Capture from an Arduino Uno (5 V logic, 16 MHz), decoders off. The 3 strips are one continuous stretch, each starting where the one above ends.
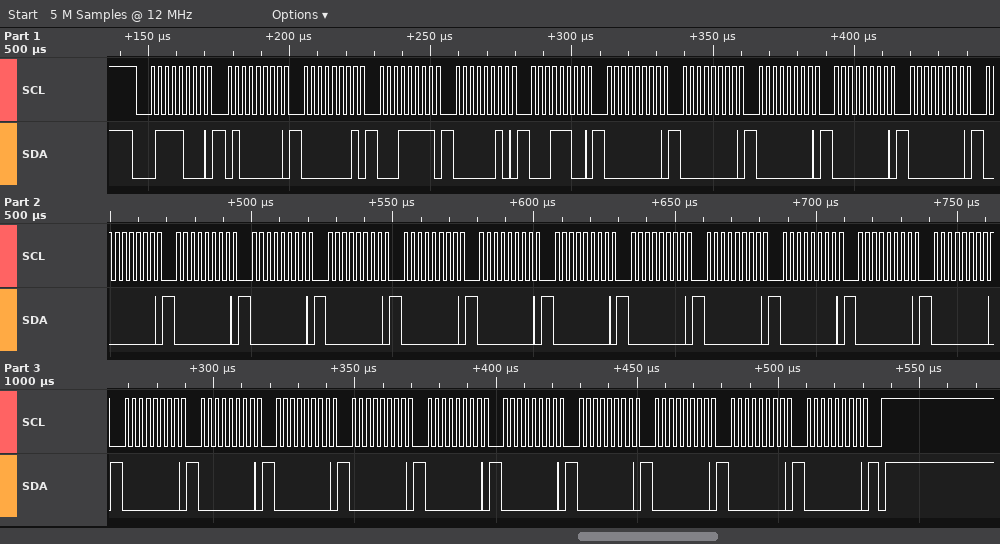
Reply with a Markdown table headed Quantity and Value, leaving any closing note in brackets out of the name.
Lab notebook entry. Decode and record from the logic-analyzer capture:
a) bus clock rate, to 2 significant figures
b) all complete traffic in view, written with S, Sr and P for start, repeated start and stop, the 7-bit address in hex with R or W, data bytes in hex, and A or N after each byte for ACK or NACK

| Quantity | Value |
|---|---|
| bus clock rate, to 2 significant figures | 400 kHz |
| all complete traffic in view, written with S, Sr and P for start, repeated start and stop, the 7-bit address in hex with R or W, data bytes in hex, and A or N after each byte for ACK or NACK | S 3CW A 40 A 01 A 1F A 02 A 1C A 00 A 00 A 00 A 00 A 00 A 00 A 00 A 00 A 00 A 00 A 00 A 00 A 00 A 00 A 00 A 00 A 00 A 00 A 00 A 00 A 00 A 00 A 00 A 00 A 00 A 00 A 00 A P |
